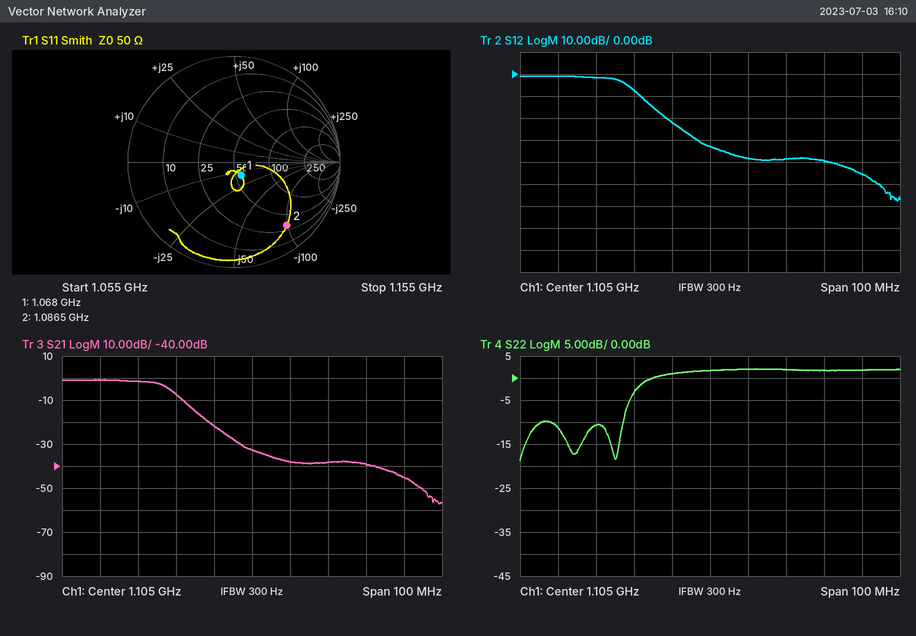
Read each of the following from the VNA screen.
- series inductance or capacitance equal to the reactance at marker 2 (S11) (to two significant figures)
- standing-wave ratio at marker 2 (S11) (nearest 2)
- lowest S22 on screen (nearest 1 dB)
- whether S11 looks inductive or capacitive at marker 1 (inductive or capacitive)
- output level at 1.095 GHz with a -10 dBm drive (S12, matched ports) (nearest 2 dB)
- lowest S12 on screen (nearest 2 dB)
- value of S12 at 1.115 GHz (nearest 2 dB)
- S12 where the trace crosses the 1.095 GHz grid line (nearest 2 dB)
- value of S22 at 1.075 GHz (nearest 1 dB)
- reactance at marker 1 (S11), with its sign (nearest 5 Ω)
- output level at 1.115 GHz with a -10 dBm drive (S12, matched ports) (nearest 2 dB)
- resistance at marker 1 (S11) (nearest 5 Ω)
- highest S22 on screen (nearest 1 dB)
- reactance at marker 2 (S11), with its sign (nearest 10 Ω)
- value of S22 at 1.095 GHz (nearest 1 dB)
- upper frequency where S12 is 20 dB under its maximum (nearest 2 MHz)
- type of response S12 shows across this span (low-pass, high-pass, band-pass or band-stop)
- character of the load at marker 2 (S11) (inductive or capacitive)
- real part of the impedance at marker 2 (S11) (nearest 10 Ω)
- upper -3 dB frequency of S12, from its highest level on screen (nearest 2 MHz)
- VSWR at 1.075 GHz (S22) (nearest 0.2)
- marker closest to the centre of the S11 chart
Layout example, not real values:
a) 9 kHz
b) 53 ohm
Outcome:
a) 1.5 pF
b) 8
c) -19 dB
d) capacitive
e) -32 dBm
f) -58 dB
g) -38 dB
h) -22 dB
i) -11 dB
j) -15 Ω
k) -48 dBm
l) 55 Ω
m) 2 dB
n) -100 Ω
o) 1 dB
p) 1.094 GHz
q) low-pass
r) capacitive
s) 30 Ω
t) 1.082 GHz
u) 1.8
v) marker 1
